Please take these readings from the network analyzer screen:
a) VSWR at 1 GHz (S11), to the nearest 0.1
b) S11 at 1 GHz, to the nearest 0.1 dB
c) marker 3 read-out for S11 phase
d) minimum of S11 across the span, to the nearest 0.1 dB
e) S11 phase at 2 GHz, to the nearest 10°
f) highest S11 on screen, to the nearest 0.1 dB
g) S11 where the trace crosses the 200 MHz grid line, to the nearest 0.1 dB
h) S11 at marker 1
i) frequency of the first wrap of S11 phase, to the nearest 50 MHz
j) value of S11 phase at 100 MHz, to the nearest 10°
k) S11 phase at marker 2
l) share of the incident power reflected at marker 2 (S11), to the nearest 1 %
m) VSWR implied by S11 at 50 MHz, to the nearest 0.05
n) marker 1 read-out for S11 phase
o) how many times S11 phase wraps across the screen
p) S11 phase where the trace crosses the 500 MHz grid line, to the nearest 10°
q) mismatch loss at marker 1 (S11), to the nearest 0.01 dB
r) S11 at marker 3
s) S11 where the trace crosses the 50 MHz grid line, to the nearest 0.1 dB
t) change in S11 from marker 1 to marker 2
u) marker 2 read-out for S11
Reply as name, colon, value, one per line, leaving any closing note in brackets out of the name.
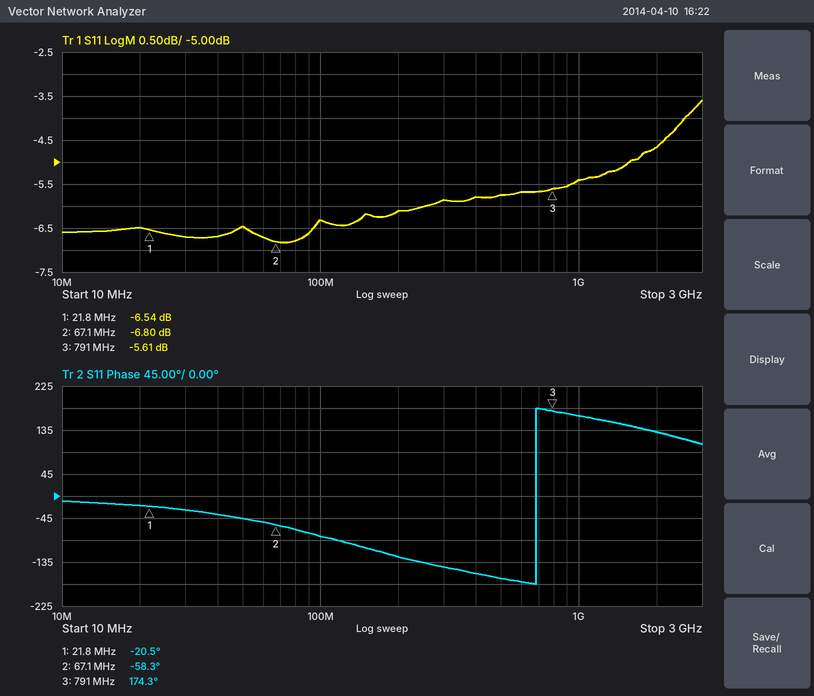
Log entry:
VSWR at 1 GHz (S11), to the nearest 0.1: 3.3
S11 at 1 GHz, to the nearest 0.1 dB: -5.4 dB
marker 3 read-out for S11 phase: 174.3°
minimum of S11 across the span, to the nearest 0.1 dB: -6.8 dB
S11 phase at 2 GHz, to the nearest 10°: 130°
highest S11 on screen, to the nearest 0.1 dB: -3.6 dB
S11 where the trace crosses the 200 MHz grid line, to the nearest 0.1 dB: -6.1 dB
S11 at marker 1: -6.54 dB
frequency of the first wrap of S11 phase, to the nearest 50 MHz: 700 MHz
value of S11 phase at 100 MHz, to the nearest 10°: -80°
S11 phase at marker 2: -58.3°
share of the incident power reflected at marker 2 (S11), to the nearest 1 %: 21 %
VSWR implied by S11 at 50 MHz, to the nearest 0.05: 2.80
marker 1 read-out for S11 phase: -20.5°
how many times S11 phase wraps across the screen: 1
S11 phase where the trace crosses the 500 MHz grid line, to the nearest 10°: -170°
mismatch loss at marker 1 (S11), to the nearest 0.01 dB: 1.09 dB
S11 at marker 3: -5.61 dB
S11 where the trace crosses the 50 MHz grid line, to the nearest 0.1 dB: -6.5 dB
change in S11 from marker 1 to marker 2: -0.26 dB
marker 2 read-out for S11: -6.80 dB
